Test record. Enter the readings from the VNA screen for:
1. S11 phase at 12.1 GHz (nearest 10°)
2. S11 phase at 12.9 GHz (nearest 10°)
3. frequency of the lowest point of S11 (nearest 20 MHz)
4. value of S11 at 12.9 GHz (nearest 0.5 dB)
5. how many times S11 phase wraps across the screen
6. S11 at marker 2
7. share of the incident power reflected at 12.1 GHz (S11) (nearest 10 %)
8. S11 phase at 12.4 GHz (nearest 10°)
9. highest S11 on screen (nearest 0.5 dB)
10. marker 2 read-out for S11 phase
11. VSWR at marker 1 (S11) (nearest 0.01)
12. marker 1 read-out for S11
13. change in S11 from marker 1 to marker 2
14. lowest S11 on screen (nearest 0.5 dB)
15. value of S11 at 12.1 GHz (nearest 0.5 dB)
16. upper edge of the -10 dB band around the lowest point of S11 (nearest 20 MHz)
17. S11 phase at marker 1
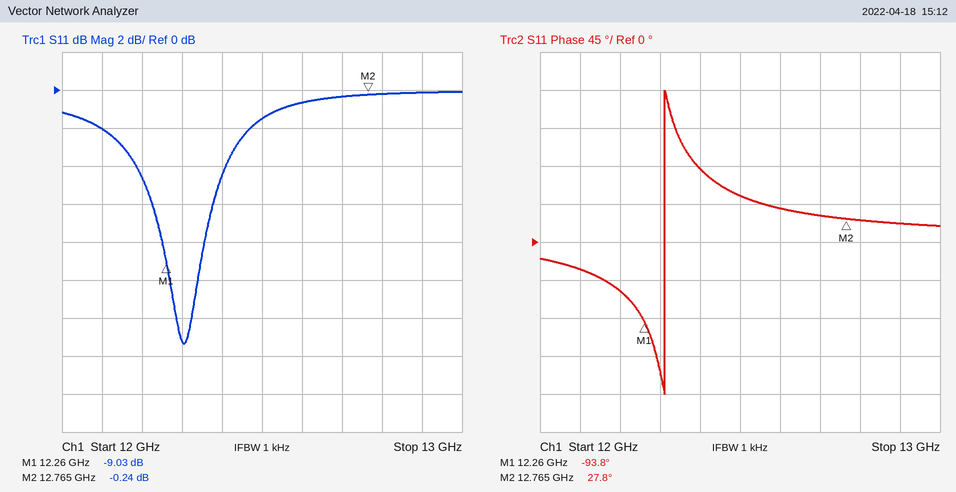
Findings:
-30°
20°
12.30 GHz
0.0 dB
1
-0.24 dB
60 %
90°
0.0 dB
27.8°
2.09
-9.03 dB
8.79 dB
-13.5 dB
-2.0 dB
12.34 GHz
-93.8°
